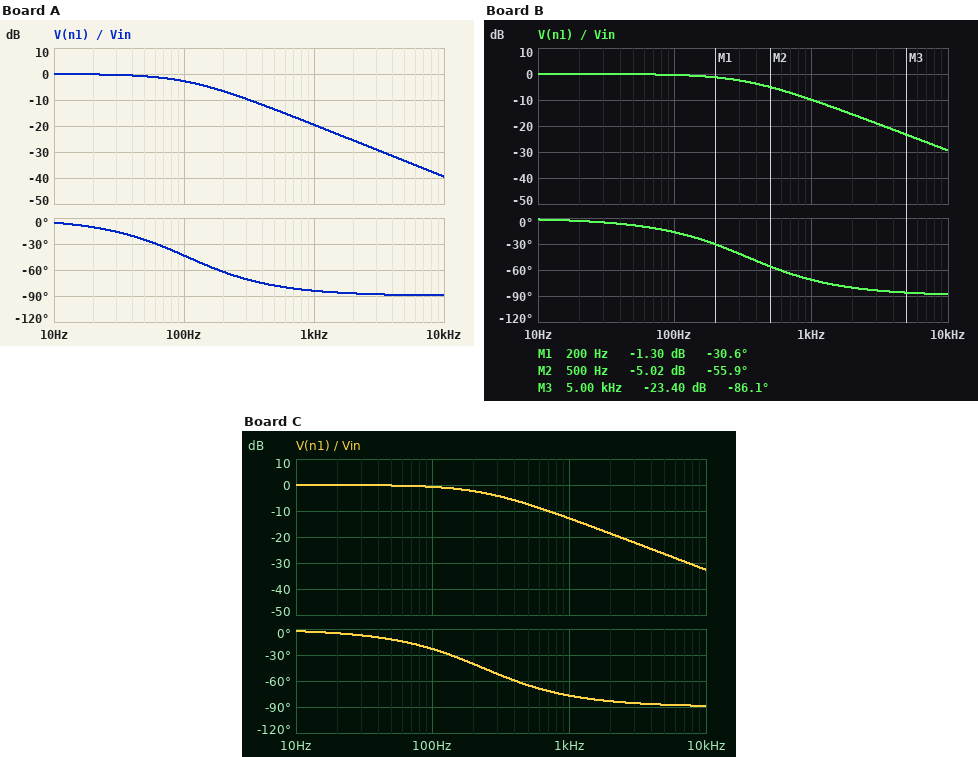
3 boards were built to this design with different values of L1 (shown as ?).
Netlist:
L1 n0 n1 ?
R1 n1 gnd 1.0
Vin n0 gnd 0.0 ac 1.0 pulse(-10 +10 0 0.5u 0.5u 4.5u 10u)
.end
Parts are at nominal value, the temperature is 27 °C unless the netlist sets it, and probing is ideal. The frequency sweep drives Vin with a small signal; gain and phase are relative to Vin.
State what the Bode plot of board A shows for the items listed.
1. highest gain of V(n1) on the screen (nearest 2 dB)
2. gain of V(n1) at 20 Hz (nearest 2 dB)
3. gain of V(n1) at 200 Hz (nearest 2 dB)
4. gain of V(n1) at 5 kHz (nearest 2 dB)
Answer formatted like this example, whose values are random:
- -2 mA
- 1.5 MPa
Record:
- 0 dB
- 0 dB
- -6 dB
- -34 dB
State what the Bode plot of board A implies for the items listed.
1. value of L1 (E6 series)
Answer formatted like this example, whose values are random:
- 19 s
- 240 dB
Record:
- 1.5 mH
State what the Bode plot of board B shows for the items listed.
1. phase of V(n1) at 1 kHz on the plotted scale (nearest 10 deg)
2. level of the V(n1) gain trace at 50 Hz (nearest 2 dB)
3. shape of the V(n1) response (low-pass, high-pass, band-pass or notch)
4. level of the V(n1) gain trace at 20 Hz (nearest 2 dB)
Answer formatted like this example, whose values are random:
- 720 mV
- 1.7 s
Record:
- -70 deg
- 0 dB
- low-pass
- 0 dB
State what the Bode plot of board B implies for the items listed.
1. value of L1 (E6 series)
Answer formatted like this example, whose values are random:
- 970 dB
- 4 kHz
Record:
- 470 µH
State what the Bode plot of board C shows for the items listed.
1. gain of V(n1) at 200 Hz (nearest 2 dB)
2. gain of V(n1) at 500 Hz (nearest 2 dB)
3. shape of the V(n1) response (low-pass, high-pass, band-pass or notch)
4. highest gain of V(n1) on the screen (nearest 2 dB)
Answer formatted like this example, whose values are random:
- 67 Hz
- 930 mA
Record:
- -2 dB
- -8 dB
- low-pass
- 0 dB
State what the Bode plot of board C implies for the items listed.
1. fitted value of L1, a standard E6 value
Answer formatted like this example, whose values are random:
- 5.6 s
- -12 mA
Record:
- 680 µH
